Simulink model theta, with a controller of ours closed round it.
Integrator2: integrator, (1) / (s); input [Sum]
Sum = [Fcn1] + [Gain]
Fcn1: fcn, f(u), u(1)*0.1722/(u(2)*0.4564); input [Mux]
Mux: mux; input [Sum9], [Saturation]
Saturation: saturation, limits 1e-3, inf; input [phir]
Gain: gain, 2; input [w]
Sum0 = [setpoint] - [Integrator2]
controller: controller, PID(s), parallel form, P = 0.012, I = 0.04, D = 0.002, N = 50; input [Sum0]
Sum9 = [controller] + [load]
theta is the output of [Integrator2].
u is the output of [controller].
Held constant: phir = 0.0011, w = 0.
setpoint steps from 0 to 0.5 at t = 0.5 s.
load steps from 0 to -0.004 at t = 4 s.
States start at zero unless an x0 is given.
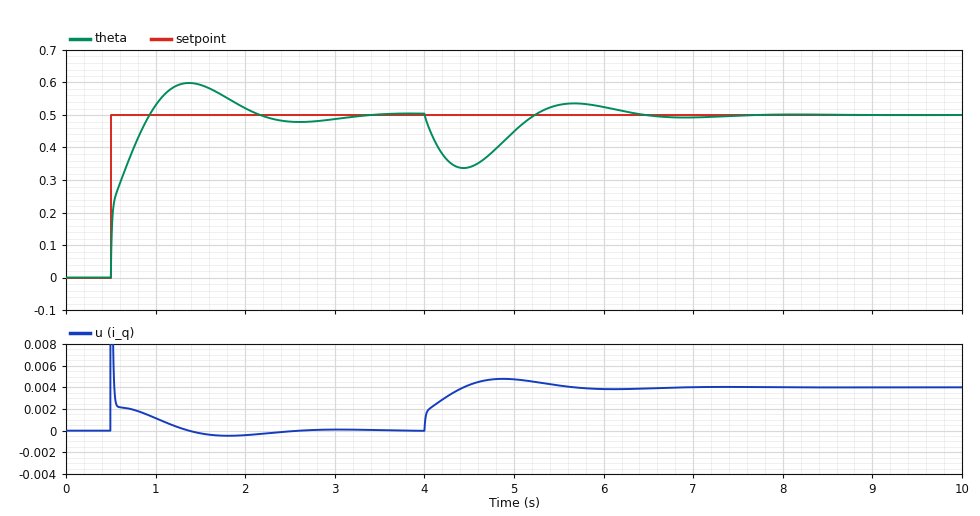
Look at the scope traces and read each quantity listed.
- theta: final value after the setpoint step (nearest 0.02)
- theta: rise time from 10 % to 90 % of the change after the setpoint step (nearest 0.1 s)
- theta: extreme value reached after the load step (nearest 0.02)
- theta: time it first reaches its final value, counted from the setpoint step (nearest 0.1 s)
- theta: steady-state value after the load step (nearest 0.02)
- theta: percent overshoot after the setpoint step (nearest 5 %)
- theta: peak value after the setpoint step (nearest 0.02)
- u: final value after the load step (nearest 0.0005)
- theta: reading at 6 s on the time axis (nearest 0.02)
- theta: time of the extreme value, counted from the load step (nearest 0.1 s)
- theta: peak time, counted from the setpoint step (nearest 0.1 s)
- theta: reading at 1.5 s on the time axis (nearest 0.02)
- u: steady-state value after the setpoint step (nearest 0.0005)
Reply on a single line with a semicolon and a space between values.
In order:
0.50; 0.3 s; 0.34; 0.4 s; 0.50; 20 %; 0.60; 0.0040; 0.52; 0.4 s; 0.9 s; 0.60; 0.0000
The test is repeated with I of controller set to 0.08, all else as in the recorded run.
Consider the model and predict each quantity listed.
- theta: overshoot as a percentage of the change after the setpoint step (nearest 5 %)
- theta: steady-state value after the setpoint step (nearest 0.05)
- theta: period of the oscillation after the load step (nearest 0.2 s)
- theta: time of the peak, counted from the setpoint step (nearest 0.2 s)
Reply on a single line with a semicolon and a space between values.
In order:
25 %; 0.50; 1.6 s; 0.6 s
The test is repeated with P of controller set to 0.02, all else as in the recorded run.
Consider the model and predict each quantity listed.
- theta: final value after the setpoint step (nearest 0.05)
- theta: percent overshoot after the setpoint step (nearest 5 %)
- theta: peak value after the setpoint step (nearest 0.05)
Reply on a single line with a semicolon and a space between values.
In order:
0.50; 10 %; 0.55
